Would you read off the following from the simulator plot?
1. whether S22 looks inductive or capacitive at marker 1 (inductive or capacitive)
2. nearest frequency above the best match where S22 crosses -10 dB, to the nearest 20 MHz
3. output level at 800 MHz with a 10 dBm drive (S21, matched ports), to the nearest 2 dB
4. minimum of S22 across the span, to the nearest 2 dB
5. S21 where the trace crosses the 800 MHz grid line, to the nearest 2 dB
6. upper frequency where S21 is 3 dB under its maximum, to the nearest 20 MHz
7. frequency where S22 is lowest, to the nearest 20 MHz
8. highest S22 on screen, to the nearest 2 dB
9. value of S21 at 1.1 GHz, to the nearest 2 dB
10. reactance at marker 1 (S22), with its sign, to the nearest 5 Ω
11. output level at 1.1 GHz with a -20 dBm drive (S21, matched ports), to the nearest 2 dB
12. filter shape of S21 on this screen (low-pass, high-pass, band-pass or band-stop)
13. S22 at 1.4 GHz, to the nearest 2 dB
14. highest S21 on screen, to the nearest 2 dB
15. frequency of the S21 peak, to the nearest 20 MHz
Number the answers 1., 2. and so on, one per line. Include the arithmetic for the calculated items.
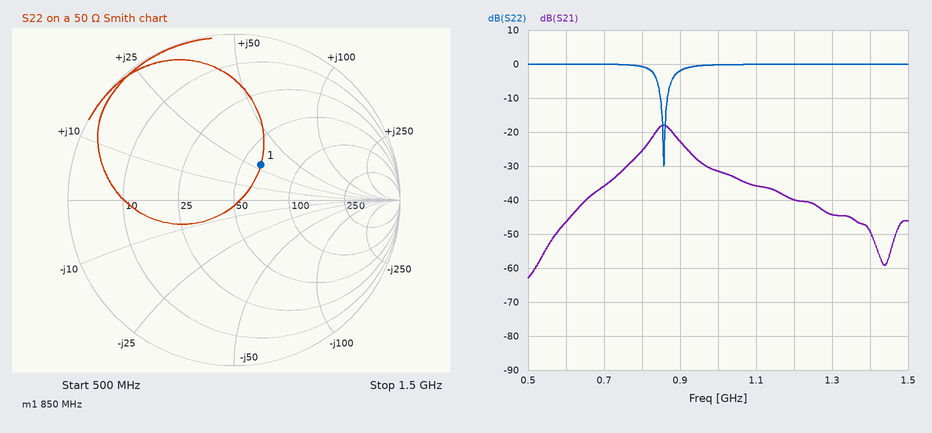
1. inductive
2. 860 MHz
3. 10 dBm + (-26 dB) = -16 dBm
4. -30 dB
5. -26 dB
6. 880 MHz
7. 860 MHz
8. 0 dB
9. -36 dB
10. +30 Ω
11. -20 dBm + (-36 dB) = -56 dBm
12. band-pass
13. 0 dB
14. -18 dB
15. 860 MHz
